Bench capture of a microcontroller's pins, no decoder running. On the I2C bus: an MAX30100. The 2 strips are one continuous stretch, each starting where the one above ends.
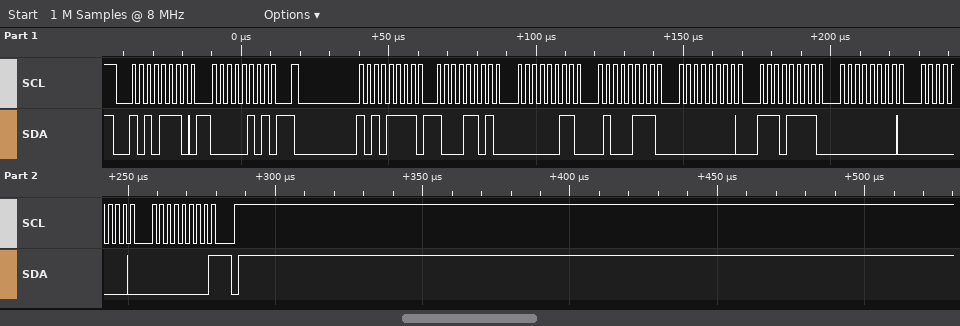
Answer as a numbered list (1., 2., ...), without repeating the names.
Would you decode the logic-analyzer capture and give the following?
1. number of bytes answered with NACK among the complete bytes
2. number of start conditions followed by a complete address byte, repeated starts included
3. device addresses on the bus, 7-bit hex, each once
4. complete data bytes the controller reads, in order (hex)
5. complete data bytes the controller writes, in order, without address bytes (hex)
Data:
1. 1
2. 2
3. 0x57
4. 8D 03 47 00 EF 00 00 00
5. 05
